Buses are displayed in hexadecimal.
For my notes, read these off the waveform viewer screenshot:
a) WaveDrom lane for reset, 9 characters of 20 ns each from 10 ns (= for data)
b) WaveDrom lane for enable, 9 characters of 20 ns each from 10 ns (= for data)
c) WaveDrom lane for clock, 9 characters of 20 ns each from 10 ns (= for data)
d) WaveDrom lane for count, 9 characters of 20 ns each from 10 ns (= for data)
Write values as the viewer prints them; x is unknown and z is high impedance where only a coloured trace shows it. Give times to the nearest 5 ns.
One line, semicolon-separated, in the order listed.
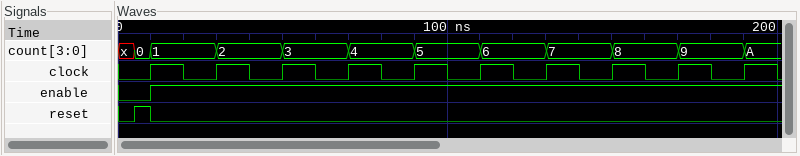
{name: 'reset', wave: '0........'}; {name: 'enable', wave: '1........'}; {name: 'clock', wave: 'p........'}; {name: 'count', wave: '=========', data: '1 2 3 4 5 6 7 8 9'}
